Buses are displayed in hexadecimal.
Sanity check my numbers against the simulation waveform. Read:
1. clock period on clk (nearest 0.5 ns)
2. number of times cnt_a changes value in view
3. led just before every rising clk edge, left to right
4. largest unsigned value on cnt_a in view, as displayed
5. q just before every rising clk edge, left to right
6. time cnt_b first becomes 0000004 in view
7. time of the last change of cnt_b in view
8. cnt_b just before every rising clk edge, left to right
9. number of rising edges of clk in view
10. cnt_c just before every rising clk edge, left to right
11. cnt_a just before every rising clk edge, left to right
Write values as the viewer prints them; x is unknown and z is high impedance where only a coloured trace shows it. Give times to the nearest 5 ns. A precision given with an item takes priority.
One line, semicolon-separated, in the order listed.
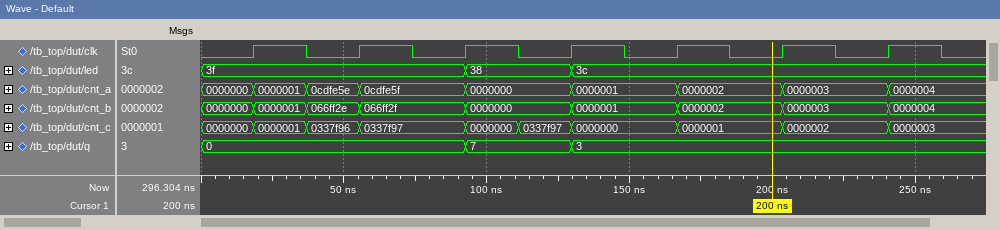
37 ns; 8; 3f, 3f, 3f, 38, 3c, 3c, 3c; 0cdfe5f; 0, 0, 0, 7, 3, 3, 3; 240 ns; 240 ns; 0000000, 066ff2e, 066ff2f, 0000000, 0000001, 0000002, 0000003; 7; 0000000, 0337f96, 0337f97, 0337f97, 0000000, 0000001, 0000002; 0000000, 0cdfe5e, 0cdfe5f, 0000000, 0000001, 0000002, 0000003
